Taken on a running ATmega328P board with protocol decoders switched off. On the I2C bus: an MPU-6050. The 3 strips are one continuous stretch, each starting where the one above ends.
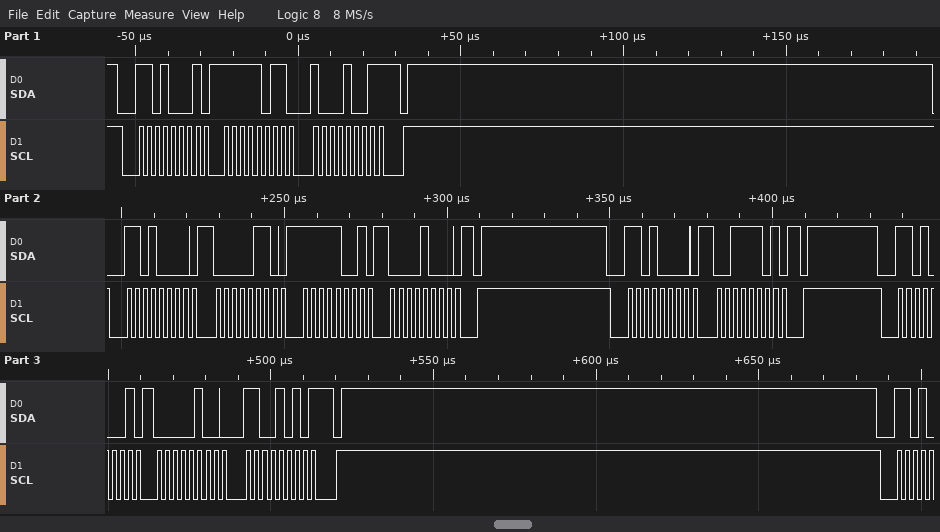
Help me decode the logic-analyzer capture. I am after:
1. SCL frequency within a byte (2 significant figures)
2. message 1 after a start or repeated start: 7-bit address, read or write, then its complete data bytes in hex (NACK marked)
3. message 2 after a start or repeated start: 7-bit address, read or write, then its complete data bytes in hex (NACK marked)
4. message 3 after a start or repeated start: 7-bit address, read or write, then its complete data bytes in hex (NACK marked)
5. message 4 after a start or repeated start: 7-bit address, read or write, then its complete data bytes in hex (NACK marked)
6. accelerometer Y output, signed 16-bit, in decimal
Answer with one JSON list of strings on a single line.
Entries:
["400 kHz", "0x68 read: FB 89 NACK", "0x68 write: 06 F9 08", "0x68 write: 3D", "0x68 read: 04 CA NACK", "1226"]
